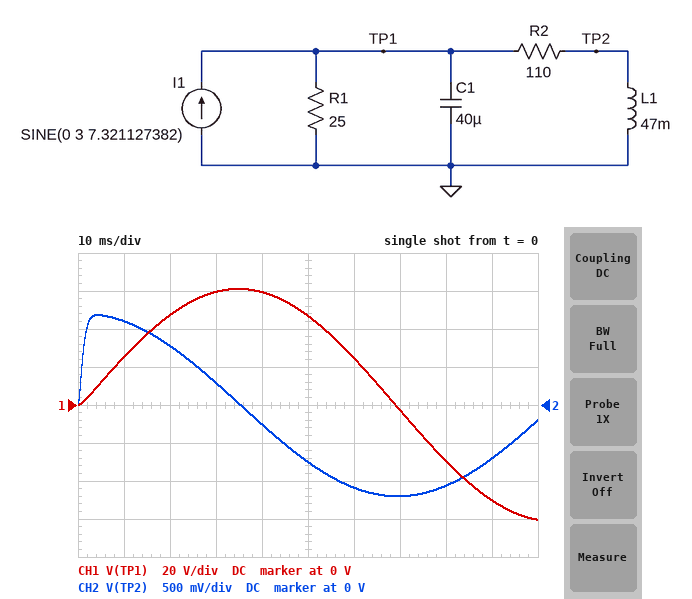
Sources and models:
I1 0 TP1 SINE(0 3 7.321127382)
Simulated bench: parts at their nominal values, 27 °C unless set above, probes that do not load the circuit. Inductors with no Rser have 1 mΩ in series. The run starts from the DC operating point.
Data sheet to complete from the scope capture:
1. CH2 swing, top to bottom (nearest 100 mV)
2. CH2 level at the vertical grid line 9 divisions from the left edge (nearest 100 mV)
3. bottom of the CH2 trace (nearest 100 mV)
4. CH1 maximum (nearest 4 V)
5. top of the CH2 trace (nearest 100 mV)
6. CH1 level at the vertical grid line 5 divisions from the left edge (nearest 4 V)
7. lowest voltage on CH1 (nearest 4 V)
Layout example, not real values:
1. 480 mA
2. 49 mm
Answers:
1. 2.4 V
2. -700 mV
3. -1.2 V
4. 60 V
5. 1.2 V
6. 48 V
7. -60 V
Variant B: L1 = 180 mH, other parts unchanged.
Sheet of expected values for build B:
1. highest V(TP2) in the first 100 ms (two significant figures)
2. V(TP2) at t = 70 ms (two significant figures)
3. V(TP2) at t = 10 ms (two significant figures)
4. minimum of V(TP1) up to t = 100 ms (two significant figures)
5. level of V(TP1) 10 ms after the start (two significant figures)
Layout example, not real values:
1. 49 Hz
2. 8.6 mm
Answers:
1. 4.5 V
2. -4.6 V
3. 4.3 V
4. -61 V
5. 26 V
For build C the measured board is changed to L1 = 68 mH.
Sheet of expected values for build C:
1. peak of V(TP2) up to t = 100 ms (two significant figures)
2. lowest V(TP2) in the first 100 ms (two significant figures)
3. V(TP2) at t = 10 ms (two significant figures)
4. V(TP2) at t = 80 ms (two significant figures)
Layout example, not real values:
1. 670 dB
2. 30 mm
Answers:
1. 1.7 V
2. -1.7 V
3. 1.6 V
4. -1.5 V
